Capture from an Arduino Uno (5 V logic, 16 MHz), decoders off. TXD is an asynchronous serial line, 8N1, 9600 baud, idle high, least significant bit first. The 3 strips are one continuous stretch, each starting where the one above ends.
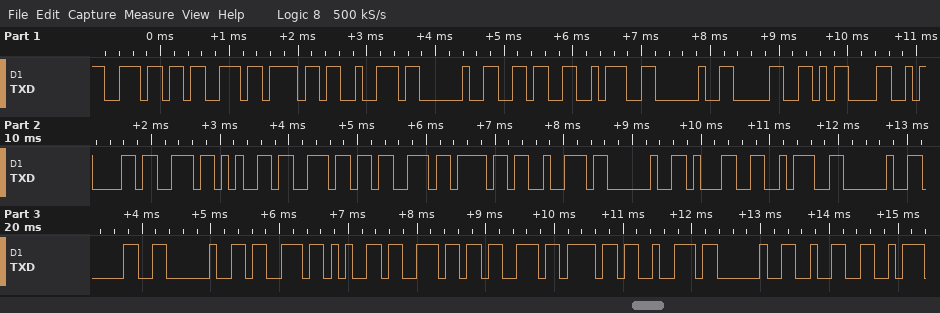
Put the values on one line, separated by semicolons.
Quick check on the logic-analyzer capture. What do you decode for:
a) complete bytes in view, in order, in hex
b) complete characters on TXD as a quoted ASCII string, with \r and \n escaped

6E 73 6F 72 20 36 3A 20 30 0D 0A 73 65 6E 73 6F 72 20 31 3A 20 30 20 73 65 6E 73 6F 72 20 32; "nsor 6: 0\r\nsensor 1: 0 sensor 2"
